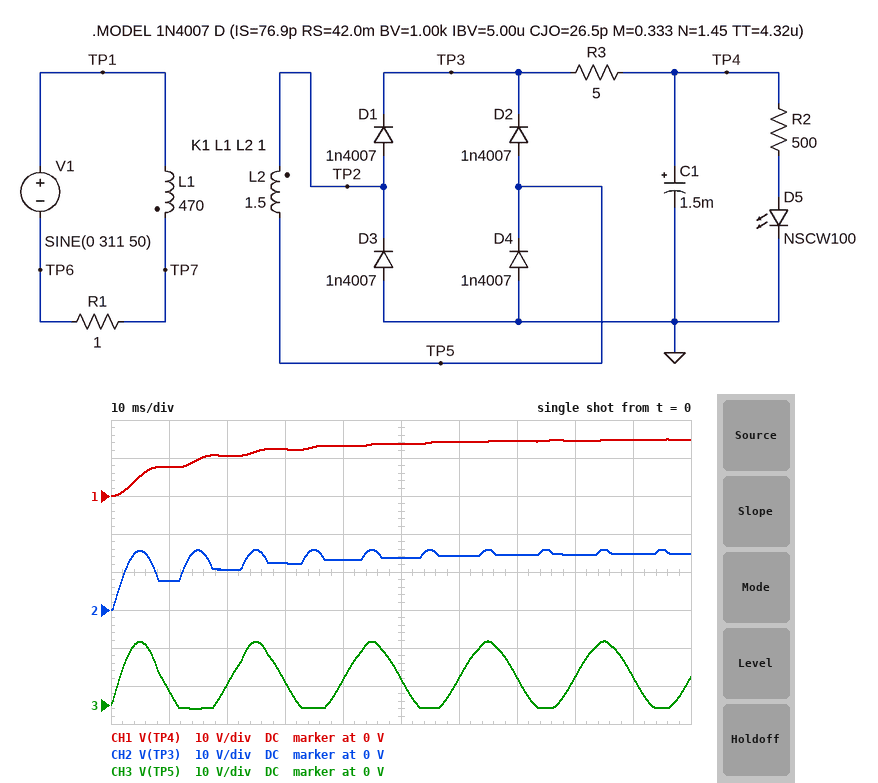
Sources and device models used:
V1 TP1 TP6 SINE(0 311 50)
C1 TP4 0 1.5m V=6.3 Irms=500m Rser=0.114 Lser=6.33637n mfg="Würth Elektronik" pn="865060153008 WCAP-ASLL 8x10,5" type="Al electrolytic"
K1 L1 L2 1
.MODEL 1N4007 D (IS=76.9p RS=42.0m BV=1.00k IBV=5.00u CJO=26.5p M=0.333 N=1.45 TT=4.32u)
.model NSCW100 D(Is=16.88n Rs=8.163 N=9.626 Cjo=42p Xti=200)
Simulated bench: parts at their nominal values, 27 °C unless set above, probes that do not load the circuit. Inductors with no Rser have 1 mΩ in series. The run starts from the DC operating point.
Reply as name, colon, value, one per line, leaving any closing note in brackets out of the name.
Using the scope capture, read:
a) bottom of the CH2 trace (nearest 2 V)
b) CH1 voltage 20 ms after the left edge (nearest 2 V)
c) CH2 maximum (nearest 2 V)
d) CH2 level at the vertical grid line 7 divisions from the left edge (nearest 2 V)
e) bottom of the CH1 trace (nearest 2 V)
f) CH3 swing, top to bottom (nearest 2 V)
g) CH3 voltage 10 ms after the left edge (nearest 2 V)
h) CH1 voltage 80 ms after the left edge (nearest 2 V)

bottom of the CH2 trace: 0 V
CH1 voltage 20 ms after the left edge: 10 V
CH2 maximum: 16 V
CH2 level at the vertical grid line 7 divisions from the left edge: 14 V
bottom of the CH1 trace: 0 V
CH3 swing, top to bottom: 18 V
CH3 voltage 10 ms after the left edge: 4 V
CH1 voltage 80 ms after the left edge: 14 V
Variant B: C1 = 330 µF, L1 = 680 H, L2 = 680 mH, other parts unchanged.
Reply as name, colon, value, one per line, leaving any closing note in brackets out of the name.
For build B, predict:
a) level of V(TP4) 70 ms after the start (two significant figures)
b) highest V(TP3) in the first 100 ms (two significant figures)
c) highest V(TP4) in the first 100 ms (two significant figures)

level of V(TP4) 70 ms after the start: 7.9 V
highest V(TP3) in the first 100 ms: 8.3 V
highest V(TP4) in the first 100 ms: 8.0 V
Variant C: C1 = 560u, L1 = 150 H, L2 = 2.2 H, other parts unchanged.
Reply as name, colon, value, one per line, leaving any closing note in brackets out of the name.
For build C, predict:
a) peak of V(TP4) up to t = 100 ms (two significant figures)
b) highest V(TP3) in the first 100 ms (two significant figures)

peak of V(TP4) up to t = 100 ms: 34 V
highest V(TP3) in the first 100 ms: 36 V
